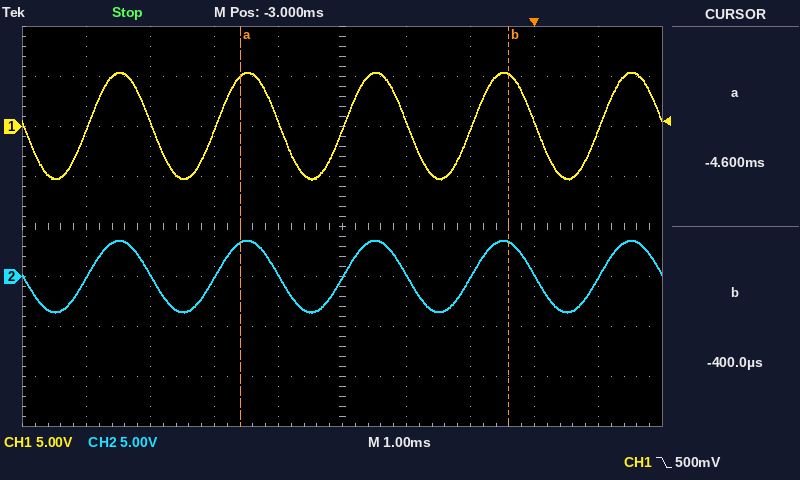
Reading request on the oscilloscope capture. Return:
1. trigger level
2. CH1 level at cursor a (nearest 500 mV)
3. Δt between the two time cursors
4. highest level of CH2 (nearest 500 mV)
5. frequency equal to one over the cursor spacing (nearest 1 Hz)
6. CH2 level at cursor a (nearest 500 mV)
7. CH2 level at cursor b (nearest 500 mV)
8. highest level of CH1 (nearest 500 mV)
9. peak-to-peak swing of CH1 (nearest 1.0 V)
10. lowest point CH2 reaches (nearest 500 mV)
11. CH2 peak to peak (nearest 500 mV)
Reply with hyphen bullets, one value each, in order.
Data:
- 500 mV
- 5.0 V
- 4.2 ms
- 3.5 V
- 238 Hz
- 3.5 V
- 3.5 V
- 5.5 V
- 11.0 V
- -3.5 V
- 7.0 V
